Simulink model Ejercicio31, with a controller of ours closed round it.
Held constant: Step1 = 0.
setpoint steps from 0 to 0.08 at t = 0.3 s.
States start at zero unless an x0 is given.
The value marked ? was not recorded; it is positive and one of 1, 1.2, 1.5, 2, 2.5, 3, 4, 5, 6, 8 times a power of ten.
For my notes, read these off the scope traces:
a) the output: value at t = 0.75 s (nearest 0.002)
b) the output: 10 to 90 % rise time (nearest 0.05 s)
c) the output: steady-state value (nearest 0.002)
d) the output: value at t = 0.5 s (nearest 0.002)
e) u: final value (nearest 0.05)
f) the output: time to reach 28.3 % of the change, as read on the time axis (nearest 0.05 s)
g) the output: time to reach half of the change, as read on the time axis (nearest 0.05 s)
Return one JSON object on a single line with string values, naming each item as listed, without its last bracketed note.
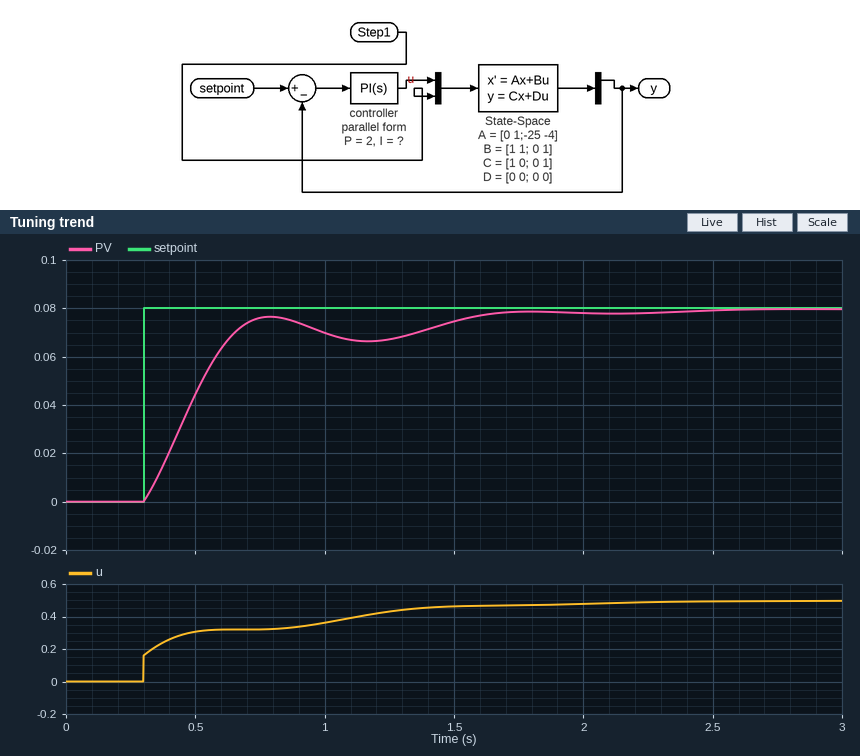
{"the output: value at t = 0.75 s": "0.076", "the output: 10 to 90 % rise time": "0.35 s", "the output: steady-state value": "0.080", "the output: value at t = 0.5 s": "0.044", "u: final value": "0.50", "the output: time to reach 28.3 % of the change, as read on the time axis": "0.40 s", "the output: time to reach half of the change, as read on the time axis": "0.50 s"}
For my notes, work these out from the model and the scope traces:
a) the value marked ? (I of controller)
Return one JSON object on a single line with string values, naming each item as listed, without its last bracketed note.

{"the value marked ?": "20"}
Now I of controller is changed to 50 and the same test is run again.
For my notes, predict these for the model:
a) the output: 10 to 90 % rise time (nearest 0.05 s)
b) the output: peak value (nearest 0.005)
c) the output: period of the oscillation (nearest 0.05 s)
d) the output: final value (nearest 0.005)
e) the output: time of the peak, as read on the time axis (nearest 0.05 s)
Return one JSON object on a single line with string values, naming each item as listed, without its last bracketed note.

{"the output: 10 to 90 % rise time": "0.15 s", "the output: peak value": "0.100", "the output: period of the oscillation": "0.75 s", "the output: final value": "0.080", "the output: time of the peak, as read on the time axis": "0.65 s"}
